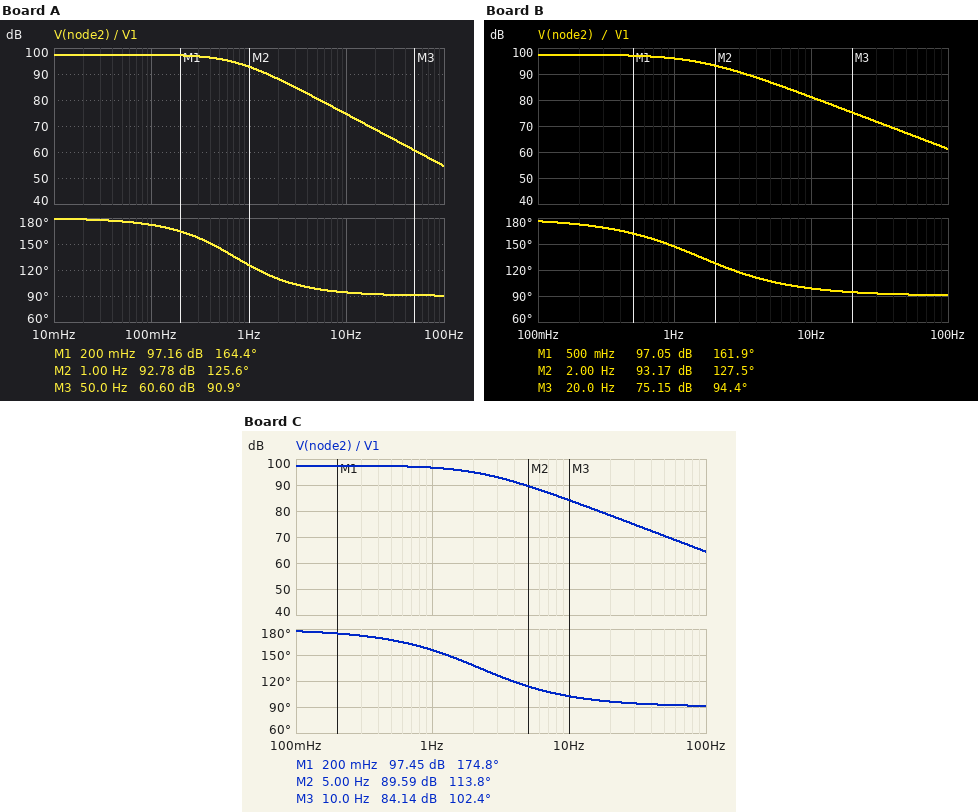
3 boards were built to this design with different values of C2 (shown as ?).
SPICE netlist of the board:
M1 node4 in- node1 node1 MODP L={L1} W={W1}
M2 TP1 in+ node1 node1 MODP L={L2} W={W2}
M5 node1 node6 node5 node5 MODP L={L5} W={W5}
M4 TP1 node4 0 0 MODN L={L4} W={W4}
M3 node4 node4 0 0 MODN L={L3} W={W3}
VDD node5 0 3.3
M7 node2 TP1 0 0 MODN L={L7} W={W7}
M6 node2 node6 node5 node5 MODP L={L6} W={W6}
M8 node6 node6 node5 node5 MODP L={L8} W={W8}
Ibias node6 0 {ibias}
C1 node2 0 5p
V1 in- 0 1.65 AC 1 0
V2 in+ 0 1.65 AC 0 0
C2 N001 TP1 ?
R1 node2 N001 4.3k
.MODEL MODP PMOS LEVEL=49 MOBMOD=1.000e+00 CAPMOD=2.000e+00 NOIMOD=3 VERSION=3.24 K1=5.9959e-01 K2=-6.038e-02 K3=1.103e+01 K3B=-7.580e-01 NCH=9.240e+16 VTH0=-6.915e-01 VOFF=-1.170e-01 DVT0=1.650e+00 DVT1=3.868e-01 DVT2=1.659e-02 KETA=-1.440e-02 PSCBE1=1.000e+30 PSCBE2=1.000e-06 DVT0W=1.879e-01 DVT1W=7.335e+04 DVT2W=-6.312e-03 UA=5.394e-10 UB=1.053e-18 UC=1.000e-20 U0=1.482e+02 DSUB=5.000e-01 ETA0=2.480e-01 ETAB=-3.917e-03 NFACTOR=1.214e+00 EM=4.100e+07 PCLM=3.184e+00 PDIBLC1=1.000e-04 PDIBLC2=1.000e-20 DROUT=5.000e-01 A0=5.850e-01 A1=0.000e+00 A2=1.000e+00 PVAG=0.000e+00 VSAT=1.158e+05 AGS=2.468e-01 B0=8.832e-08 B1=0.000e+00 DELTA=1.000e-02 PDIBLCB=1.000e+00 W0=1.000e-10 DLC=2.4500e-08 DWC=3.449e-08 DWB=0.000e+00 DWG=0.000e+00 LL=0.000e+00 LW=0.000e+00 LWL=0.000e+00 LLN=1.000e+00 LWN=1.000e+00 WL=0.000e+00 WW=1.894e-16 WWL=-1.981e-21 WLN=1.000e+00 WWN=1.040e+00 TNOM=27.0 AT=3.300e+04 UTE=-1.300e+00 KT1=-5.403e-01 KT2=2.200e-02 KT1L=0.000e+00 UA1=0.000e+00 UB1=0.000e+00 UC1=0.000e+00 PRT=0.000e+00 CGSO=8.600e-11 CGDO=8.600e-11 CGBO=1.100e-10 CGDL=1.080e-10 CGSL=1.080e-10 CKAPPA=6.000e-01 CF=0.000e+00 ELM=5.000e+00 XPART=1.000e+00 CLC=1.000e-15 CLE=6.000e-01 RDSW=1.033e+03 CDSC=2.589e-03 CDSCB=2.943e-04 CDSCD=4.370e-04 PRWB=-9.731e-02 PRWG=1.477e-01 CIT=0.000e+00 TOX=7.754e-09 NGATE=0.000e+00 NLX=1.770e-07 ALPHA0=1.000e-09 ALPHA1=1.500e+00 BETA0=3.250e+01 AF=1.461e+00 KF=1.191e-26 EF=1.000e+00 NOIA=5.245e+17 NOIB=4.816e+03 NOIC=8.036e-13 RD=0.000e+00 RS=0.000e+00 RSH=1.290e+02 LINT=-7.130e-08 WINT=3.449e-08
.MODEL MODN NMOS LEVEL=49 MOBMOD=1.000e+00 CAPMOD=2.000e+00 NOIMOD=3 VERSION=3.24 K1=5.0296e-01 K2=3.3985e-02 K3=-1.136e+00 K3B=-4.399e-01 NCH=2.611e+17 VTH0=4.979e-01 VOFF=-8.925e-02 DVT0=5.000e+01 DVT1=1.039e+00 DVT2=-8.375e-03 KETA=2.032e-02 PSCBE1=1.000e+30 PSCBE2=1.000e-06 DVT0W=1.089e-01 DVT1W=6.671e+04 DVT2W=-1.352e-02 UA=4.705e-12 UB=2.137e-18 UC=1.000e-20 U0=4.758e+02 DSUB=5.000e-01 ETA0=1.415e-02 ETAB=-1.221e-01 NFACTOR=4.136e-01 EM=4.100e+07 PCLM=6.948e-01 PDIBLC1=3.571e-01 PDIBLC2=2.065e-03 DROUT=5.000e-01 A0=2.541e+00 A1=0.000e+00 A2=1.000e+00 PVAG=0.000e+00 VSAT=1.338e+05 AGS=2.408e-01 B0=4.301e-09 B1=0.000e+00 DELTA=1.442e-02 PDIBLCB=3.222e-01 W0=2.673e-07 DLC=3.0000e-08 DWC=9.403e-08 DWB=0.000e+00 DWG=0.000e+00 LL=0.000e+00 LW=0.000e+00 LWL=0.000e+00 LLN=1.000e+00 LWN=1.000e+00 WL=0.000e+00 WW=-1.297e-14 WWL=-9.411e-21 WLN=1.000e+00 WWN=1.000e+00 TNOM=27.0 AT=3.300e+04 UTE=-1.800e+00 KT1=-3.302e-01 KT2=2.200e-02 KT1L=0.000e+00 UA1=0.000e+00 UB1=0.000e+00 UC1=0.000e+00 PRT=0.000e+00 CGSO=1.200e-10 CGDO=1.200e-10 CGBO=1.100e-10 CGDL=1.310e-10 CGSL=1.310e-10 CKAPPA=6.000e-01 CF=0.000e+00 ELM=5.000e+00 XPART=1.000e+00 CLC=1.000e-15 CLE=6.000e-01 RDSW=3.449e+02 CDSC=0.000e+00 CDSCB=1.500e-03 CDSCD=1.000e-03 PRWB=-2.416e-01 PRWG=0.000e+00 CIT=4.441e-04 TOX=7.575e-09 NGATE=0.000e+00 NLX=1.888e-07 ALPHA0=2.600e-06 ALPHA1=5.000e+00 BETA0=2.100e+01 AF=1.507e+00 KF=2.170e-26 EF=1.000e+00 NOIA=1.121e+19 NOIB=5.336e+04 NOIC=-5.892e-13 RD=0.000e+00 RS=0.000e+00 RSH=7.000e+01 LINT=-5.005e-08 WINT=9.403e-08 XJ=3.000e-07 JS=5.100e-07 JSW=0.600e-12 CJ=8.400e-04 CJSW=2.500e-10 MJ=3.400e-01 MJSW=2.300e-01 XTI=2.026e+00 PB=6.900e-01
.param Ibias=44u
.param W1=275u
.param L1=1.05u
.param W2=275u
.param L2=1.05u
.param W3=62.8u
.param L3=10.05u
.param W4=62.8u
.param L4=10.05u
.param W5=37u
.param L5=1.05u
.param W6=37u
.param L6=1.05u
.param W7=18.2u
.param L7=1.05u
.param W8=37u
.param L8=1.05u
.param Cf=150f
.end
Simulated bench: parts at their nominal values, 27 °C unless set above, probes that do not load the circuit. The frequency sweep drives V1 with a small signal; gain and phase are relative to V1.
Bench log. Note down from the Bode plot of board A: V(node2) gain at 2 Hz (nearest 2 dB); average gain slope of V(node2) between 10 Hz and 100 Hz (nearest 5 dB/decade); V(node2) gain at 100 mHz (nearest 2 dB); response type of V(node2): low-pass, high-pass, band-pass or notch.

88 dB
-20 dB/decade
98 dB
low-pass
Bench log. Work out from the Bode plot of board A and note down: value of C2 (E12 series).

1.2 nF
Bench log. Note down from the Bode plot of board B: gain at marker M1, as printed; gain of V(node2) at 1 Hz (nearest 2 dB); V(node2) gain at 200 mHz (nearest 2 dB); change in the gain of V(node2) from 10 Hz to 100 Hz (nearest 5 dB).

97.05 dB
96 dB
98 dB
-20 dB
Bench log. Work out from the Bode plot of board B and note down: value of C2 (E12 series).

560 pF
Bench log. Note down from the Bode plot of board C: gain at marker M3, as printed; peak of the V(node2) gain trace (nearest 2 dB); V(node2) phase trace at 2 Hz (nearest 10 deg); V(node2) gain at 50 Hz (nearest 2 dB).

84.14 dB
98 dB
140 deg
70 dB
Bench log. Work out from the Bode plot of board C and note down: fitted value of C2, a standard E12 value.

390 pF
